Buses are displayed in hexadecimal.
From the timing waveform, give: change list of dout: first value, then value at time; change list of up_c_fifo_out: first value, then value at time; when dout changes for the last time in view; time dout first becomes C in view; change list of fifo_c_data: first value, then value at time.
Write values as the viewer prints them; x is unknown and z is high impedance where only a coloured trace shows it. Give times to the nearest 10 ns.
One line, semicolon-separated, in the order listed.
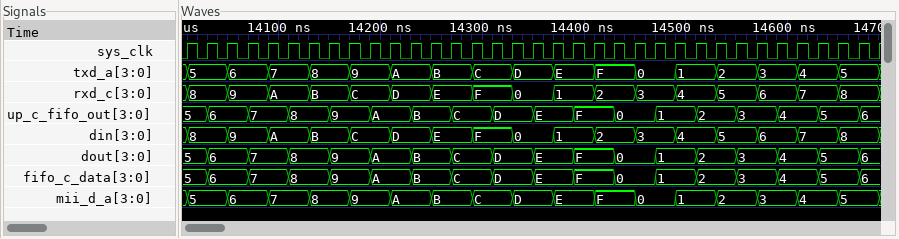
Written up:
5, 6 at 14030 ns, 7 at 14070 ns, 8 at 14110 ns, 9 at 14150 ns, A at 14190 ns, B at 14230 ns, C at 14270 ns, D at 14310 ns, E at 14350 ns, F at 14390 ns, 0 at 14430 ns, 1 at 14470 ns, 2 at 14510 ns, 3 at 14550 ns, 4 at 14590 ns, 5 at 14630 ns, 6 at 14670 ns; 5, 6 at 14030 ns, 7 at 14070 ns, 8 at 14110 ns, 9 at 14150 ns, A at 14190 ns, B at 14230 ns, C at 14270 ns, D at 14310 ns, E at 14350 ns, F at 14390 ns, 0 at 14430 ns, 1 at 14470 ns, 2 at 14510 ns, 3 at 14550 ns, 4 at 14590 ns, 5 at 14630 ns, 6 at 14670 ns; 14670 ns; 14270 ns; 5, 6 at 14030 ns, 7 at 14070 ns, 8 at 14110 ns, 9 at 14150 ns, A at 14190 ns, B at 14230 ns, C at 14270 ns, D at 14310 ns, E at 14350 ns, F at 14390 ns, 0 at 14430 ns, 1 at 14470 ns, 2 at 14510 ns, 3 at 14550 ns, 4 at 14590 ns, 5 at 14630 ns, 6 at 14670 ns
